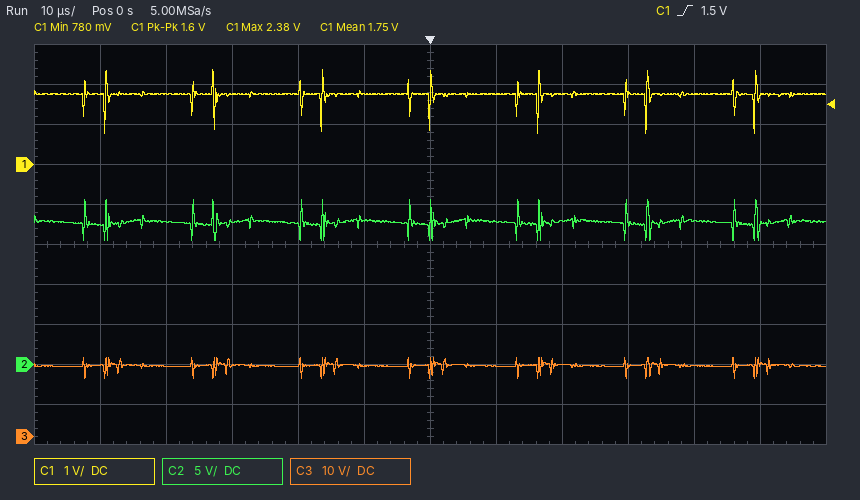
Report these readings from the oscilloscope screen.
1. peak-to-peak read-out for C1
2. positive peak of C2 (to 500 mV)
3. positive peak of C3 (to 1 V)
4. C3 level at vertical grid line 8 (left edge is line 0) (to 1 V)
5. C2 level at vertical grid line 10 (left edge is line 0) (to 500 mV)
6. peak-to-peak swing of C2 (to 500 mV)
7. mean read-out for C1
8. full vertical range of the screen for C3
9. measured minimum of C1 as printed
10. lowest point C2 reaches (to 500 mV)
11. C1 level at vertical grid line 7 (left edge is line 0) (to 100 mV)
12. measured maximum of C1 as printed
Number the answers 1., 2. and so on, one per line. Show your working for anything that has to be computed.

1. 1.6 V
2. 20.5 V
3. 20 V
4. 18 V
5. 18.0 V
6. 20.5 V − (15.5 V) = 5.0 V
7. 1.75 V
8. 100 V
9. 780 mV
10. 15.5 V
11. 1.8 V
12. 2.38 V
